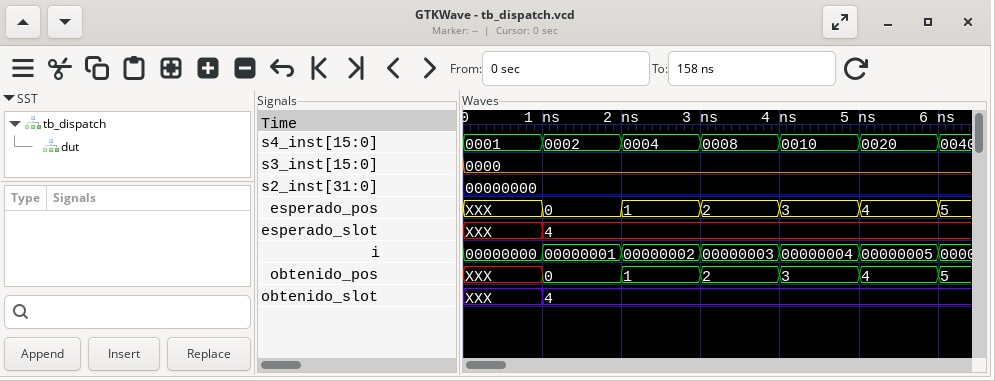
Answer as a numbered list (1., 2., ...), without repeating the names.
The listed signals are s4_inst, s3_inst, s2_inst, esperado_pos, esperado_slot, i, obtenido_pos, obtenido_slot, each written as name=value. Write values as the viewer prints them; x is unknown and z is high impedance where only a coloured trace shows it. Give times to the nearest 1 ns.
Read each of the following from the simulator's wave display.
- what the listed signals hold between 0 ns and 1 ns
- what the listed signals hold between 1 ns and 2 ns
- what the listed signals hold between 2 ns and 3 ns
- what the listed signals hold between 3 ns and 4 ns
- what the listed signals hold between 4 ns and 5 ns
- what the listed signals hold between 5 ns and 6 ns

1. s4_inst=0001, s3_inst=0000, s2_inst=00000000, esperado_pos=XXX, esperado_slot=XXX, i=00000000, obtenido_pos=XXX, obtenido_slot=XXX
2. s4_inst=0002, s3_inst=0000, s2_inst=00000000, esperado_pos=0, esperado_slot=4, i=00000001, obtenido_pos=0, obtenido_slot=4
3. s4_inst=0004, s3_inst=0000, s2_inst=00000000, esperado_pos=1, esperado_slot=4, i=00000002, obtenido_pos=1, obtenido_slot=4
4. s4_inst=0008, s3_inst=0000, s2_inst=00000000, esperado_pos=2, esperado_slot=4, i=00000003, obtenido_pos=2, obtenido_slot=4
5. s4_inst=0010, s3_inst=0000, s2_inst=00000000, esperado_pos=3, esperado_slot=4, i=00000004, obtenido_pos=3, obtenido_slot=4
6. s4_inst=0020, s3_inst=0000, s2_inst=00000000, esperado_pos=4, esperado_slot=4, i=00000005, obtenido_pos=4, obtenido_slot=4
